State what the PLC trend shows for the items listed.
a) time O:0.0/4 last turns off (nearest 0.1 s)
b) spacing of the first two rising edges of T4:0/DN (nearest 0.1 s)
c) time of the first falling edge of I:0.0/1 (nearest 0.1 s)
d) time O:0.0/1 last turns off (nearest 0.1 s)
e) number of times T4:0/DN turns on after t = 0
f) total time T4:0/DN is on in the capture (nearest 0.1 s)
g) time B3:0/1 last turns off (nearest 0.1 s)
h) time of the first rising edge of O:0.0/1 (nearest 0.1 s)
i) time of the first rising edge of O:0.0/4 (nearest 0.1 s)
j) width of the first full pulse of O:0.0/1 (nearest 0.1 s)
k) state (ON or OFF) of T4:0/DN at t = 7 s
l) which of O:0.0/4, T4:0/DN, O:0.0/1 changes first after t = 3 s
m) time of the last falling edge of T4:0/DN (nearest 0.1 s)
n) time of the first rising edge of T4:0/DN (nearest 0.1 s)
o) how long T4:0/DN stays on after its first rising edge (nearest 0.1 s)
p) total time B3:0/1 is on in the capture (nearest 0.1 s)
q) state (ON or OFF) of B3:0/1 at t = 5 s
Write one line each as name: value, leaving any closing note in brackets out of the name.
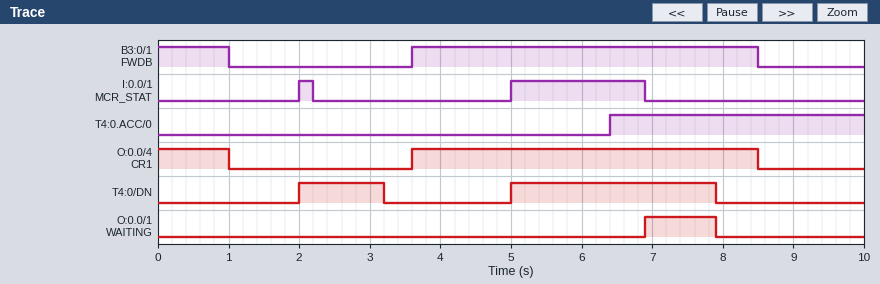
time O:0.0/4 last turns off: 8.5 s
spacing of the first two rising edges of T4:0/DN: 3.0 s
time of the first falling edge of I:0.0/1: 2.2 s
time O:0.0/1 last turns off: 7.9 s
number of times T4:0/DN turns on after t = 0: 2
total time T4:0/DN is on in the capture: 4.1 s
time B3:0/1 last turns off: 8.5 s
time of the first rising edge of O:0.0/1: 6.9 s
time of the first rising edge of O:0.0/4: 3.6 s
width of the first full pulse of O:0.0/1: 1.0 s
state (ON or OFF) of T4:0/DN at t = 7 s: ON
which of O:0.0/4, T4:0/DN, O:0.0/1 changes first after t = 3 s: T4:0/DN
time of the last falling edge of T4:0/DN: 7.9 s
time of the first rising edge of T4:0/DN: 2.0 s
how long T4:0/DN stays on after its first rising edge: 1.2 s
total time B3:0/1 is on in the capture: 5.9 s
state (ON or OFF) of B3:0/1 at t = 5 s: ON
